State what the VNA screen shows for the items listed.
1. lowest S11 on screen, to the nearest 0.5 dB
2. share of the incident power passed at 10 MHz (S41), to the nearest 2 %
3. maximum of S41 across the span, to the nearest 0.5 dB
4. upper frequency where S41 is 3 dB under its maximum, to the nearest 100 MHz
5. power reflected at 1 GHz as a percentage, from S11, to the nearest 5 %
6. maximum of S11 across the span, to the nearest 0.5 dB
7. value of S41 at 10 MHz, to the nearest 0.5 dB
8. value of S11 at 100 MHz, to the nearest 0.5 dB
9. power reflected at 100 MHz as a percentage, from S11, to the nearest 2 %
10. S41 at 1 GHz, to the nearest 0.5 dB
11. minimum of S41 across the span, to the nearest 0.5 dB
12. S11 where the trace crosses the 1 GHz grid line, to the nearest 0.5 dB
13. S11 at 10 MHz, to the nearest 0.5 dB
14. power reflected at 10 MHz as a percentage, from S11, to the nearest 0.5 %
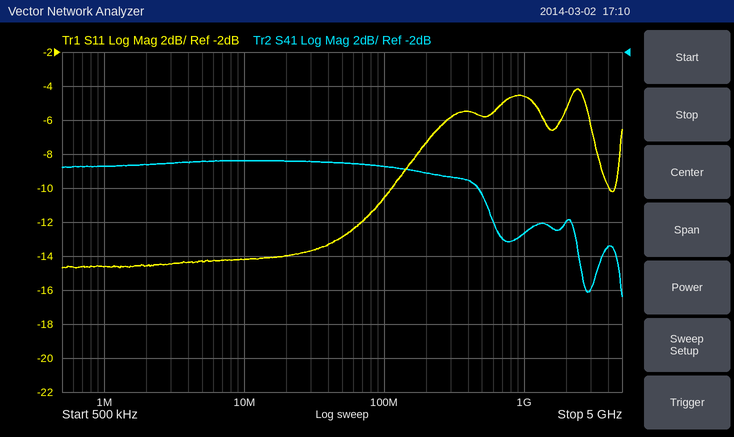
-14.5 dB
14 %
-8.5 dB
600 MHz
35 %
-4.0 dB
-8.5 dB
-10.5 dB
8 %
-12.5 dB
-16.5 dB
-4.5 dB
-14.0 dB
4.0 %
